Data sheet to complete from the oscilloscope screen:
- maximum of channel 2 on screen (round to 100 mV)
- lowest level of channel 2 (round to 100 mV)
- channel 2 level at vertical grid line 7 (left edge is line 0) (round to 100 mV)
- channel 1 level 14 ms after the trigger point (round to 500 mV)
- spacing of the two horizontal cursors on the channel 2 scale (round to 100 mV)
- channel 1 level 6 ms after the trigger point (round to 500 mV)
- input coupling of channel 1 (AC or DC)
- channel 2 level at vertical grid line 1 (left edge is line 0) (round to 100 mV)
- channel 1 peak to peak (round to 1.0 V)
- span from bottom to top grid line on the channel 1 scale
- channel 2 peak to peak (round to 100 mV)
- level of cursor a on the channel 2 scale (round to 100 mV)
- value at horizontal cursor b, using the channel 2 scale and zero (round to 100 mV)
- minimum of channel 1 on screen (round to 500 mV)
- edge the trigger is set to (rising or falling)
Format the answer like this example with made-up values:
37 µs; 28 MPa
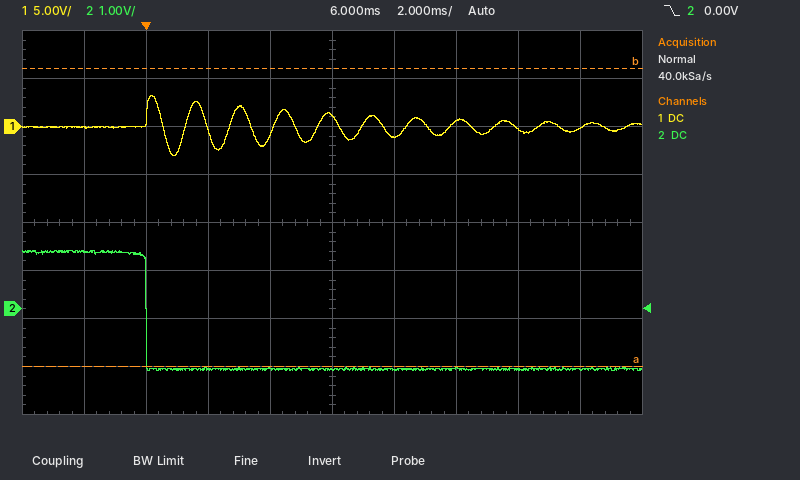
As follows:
1.2 V; -1.3 V; -1.2 V; 0.0 V; 6.2 V; 1.0 V; DC; 1.2 V; 6.0 V; 40 V; 2.5 V; -1.2 V; 5.0 V; -3.0 V; falling
